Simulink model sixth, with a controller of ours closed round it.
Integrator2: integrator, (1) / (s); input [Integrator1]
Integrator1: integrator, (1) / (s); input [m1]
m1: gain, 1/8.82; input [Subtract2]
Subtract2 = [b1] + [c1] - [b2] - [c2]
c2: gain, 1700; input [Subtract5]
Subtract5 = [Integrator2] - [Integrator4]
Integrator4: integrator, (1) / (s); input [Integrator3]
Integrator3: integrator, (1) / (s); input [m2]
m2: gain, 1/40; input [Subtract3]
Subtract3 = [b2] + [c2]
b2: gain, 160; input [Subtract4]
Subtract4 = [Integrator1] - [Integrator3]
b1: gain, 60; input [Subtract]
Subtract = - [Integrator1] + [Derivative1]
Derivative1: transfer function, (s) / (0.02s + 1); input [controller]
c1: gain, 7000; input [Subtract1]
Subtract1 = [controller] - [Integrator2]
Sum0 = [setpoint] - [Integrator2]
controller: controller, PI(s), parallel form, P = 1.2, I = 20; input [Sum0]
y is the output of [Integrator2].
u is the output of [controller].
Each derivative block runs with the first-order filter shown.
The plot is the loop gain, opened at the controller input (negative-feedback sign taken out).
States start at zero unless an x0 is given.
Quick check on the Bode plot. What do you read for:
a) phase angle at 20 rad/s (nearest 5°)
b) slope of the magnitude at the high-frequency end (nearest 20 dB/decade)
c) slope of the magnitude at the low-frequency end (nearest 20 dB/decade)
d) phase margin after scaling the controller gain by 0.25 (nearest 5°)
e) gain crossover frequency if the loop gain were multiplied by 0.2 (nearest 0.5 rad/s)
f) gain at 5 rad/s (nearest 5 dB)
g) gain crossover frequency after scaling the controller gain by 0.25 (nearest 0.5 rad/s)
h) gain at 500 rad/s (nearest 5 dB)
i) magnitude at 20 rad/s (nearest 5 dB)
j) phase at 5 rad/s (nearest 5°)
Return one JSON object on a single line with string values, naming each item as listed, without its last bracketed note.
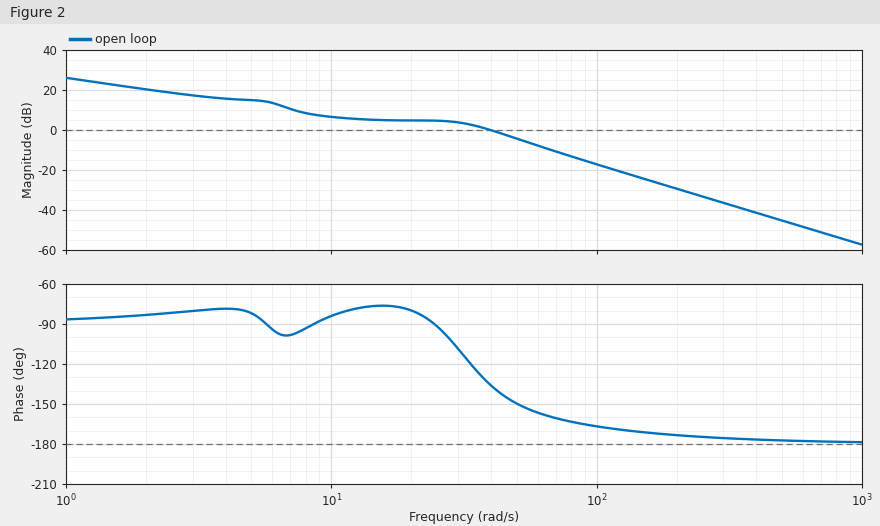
{"phase angle at 20 rad/s": "-80°", "slope of the magnitude at the high-frequency end": "-40 dB/decade", "slope of the magnitude at the low-frequency end": "-20 dB/decade", "phase margin after scaling the controller gain by 0.25": "80°", "gain crossover frequency if the loop gain were multiplied by 0.2": "6.0 rad/s", "gain at 5 rad/s": "15 dB", "gain crossover frequency after scaling the controller gain by 0.25": "6.5 rad/s", "gain at 500 rad/s": "-45 dB", "magnitude at 20 rad/s": "5 dB", "phase at 5 rad/s": "-80°"}
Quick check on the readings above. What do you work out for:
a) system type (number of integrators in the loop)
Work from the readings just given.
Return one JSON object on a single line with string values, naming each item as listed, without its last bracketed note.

{"system type": "1"}
